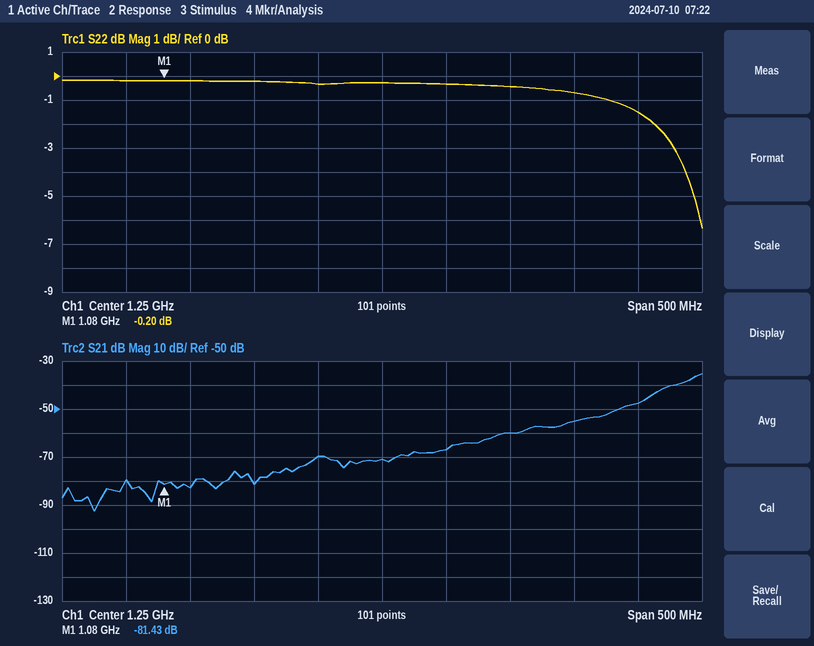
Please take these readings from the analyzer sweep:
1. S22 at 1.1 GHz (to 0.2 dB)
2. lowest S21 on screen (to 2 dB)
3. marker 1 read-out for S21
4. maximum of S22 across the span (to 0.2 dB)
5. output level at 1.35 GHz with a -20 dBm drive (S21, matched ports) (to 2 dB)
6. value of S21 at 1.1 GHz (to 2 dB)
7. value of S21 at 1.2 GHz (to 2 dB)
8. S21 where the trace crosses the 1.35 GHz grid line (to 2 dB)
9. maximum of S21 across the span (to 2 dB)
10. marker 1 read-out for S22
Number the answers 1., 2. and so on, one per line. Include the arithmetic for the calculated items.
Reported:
1. -0.2 dB
2. -92 dB
3. -81.43 dB
4. -0.2 dB
5. -20 dBm + (-60 dB) = -80 dBm
6. -82 dB
7. -70 dB
8. -60 dB
9. -36 dB
10. -0.20 dB
